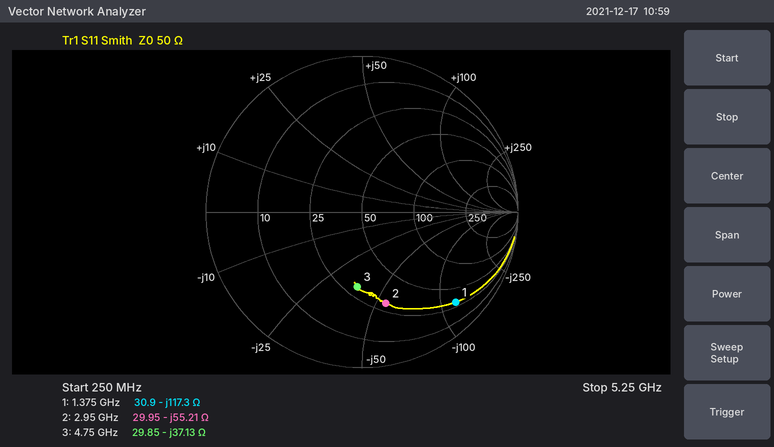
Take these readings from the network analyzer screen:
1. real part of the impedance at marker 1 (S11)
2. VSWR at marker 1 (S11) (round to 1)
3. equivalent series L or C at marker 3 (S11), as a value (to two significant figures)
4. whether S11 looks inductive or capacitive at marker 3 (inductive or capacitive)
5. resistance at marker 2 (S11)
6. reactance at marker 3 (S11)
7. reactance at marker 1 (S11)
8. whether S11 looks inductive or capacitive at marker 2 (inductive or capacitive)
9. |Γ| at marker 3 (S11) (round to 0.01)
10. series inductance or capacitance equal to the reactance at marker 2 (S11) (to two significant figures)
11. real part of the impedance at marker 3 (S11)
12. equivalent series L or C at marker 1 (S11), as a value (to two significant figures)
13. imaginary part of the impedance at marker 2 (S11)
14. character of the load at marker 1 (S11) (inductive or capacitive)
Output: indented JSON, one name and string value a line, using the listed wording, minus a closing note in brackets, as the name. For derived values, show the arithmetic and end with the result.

{
  "real part of the impedance at marker 1": "30.9 Ω",
  "VSWR at marker 1 (S11)": "11",
  "equivalent series L or C at marker 3 (S11), as a value": "C = 1/(2π × 4.75 GHz × 37.13 Ω) ≈ 902 fF, so 900 fF to two significant figures",
  "whether S11 looks inductive or capacitive at marker 3": "capacitive",
  "resistance at marker 2": "29.95 Ω",
  "reactance at marker 3": "-37.13 Ω",
  "reactance at marker 1": "-117.3 Ω",
  "whether S11 looks inductive or capacitive at marker 2": "capacitive",
  "|Γ| at marker 3 (S11)": "0.48",
  "series inductance or capacitance equal to the reactance at marker 2 (S11)": "C = 1/(2π × 2.95 GHz × 55.21 Ω) ≈ 977 fF, so 980 fF to two significant figures",
  "real part of the impedance at marker 3": "29.85 Ω",
  "equivalent series L or C at marker 1 (S11), as a value": "C = 1/(2π × 1.375 GHz × 117.3 Ω) ≈ 987 fF, so 990 fF to two significant figures",
  "imaginary part of the impedance at marker 2": "-55.21 Ω",
  "character of the load at marker 1 (S11)": "capacitive"
}
